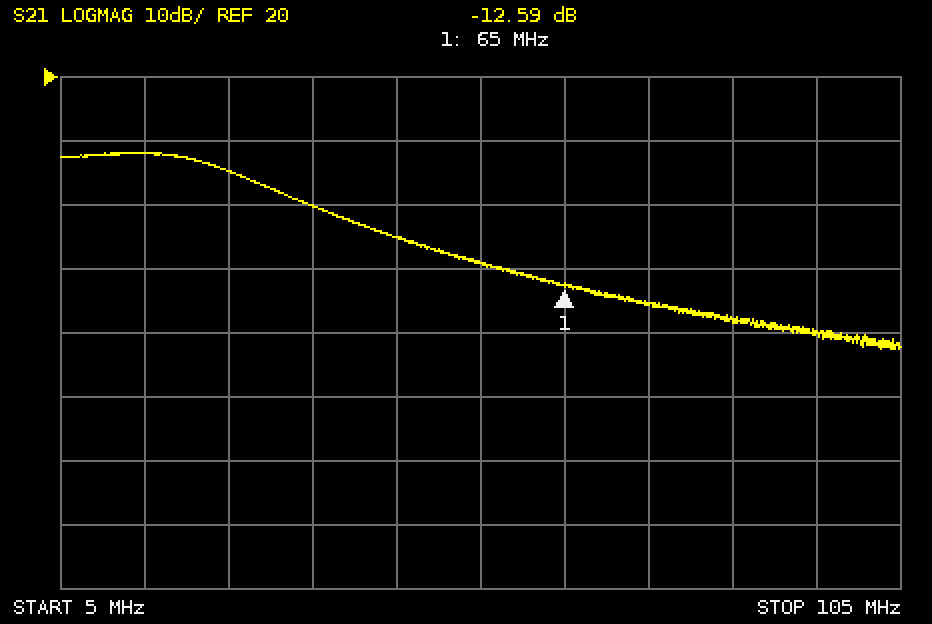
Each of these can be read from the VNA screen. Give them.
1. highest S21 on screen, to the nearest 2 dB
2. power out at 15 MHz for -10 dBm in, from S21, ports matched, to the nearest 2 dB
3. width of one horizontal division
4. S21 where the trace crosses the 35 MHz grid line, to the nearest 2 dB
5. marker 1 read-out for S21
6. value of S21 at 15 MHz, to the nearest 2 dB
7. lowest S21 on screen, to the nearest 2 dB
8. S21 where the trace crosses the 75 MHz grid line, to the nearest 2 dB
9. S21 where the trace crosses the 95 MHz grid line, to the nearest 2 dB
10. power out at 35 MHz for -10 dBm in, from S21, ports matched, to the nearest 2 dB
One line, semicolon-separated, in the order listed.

8 dB; -2 dBm; 10 MHz; 0 dB; -12.59 dB; 8 dB; -22 dB; -16 dB; -20 dB; -10 dBm
